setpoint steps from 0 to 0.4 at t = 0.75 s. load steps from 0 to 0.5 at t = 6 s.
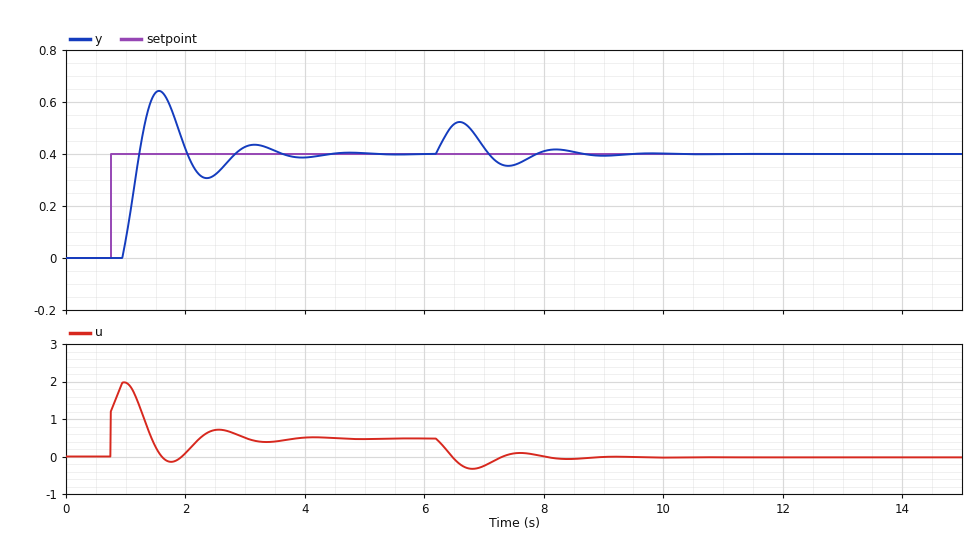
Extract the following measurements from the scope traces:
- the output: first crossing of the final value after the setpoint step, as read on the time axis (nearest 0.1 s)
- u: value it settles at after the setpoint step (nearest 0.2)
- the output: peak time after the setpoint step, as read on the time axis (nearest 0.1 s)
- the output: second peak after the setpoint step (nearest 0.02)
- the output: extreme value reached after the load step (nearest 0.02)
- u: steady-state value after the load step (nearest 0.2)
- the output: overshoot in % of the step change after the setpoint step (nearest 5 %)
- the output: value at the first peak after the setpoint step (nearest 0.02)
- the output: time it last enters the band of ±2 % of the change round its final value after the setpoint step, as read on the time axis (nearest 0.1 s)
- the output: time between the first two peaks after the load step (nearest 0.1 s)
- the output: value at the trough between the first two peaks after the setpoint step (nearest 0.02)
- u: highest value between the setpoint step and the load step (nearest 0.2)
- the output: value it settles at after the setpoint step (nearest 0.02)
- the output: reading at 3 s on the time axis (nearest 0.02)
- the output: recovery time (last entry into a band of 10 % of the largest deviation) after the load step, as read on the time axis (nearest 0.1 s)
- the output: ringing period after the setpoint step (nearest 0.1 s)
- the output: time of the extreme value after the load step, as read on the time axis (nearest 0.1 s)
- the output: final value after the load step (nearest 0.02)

1.2 s
0.4
1.6 s
0.44
0.52
0.0
60 %
0.64
4.2 s
1.6 s
0.30
2.0
0.40
0.42
8.4 s
1.6 s
6.6 s
0.40
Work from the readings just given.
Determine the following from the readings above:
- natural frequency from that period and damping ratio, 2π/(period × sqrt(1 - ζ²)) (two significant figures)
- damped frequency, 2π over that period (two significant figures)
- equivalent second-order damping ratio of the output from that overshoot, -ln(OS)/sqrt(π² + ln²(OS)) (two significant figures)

4.0 rad/s
3.9 rad/s
0.16
